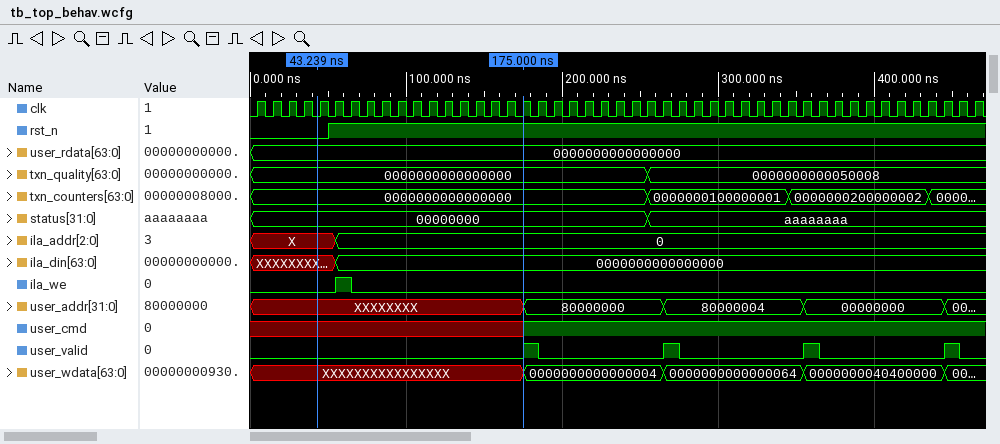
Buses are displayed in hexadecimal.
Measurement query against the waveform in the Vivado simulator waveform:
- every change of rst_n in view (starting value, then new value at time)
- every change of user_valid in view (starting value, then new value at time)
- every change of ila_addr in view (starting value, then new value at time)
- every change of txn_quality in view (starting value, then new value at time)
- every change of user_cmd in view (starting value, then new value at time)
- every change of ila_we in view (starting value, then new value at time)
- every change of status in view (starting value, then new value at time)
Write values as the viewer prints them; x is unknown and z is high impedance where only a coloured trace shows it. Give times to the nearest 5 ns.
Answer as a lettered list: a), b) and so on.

a) 0, 1 at 50 ns
b) 0, 1 at 175 ns, 0 at 185 ns, 1 at 265 ns, 0 at 275 ns, 1 at 355 ns, 0 at 365 ns, 1 at 445 ns, 0 at 455 ns
c) X, 0 at 55 ns
d) 0000000000000000, 0000000000050008 at 255 ns
e) x, 1 at 175 ns
f) 0, 1 at 55 ns, 0 at 65 ns
g) 00000000, aaaaaaaa at 255 ns
